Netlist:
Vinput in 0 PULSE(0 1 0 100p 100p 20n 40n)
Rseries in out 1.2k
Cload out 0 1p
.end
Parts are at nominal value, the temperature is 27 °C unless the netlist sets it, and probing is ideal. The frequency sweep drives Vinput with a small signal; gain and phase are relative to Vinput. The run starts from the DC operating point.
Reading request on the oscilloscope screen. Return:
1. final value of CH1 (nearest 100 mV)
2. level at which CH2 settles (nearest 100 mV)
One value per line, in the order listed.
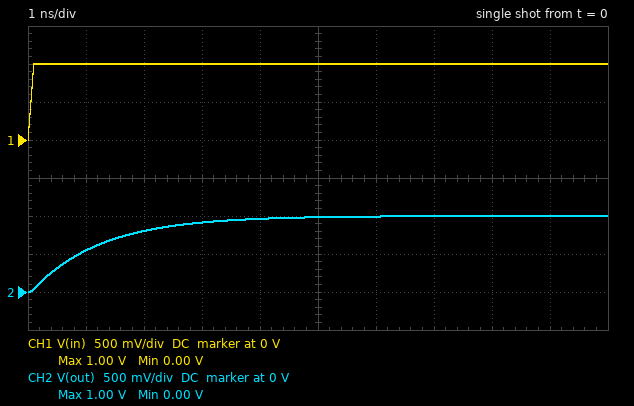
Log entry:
1.0 V
1.0 V
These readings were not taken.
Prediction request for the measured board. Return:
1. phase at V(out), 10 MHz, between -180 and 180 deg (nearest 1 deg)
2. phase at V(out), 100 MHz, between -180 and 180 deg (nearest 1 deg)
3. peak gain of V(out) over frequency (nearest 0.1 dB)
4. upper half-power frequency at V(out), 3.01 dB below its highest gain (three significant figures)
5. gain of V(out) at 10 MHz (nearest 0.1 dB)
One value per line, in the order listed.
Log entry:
-4 deg
-37 deg
0 dB
133 MHz
0 dB
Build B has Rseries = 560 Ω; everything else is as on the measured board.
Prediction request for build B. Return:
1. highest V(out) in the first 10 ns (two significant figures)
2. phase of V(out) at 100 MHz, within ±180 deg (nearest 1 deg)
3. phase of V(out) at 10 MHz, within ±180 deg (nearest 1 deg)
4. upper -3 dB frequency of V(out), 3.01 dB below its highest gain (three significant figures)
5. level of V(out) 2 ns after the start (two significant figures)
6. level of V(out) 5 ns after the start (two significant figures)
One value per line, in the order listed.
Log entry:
1.0 V
-19 deg
-2 deg
284 MHz
970 mV
1.0 V
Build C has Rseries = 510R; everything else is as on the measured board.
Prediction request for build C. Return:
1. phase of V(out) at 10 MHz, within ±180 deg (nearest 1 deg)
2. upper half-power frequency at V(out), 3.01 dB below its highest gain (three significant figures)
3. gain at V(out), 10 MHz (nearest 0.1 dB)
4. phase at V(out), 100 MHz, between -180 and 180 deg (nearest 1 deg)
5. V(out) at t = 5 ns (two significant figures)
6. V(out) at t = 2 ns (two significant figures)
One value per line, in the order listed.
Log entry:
-2 deg
312 MHz
0 dB
-18 deg
1.0 V
980 mV
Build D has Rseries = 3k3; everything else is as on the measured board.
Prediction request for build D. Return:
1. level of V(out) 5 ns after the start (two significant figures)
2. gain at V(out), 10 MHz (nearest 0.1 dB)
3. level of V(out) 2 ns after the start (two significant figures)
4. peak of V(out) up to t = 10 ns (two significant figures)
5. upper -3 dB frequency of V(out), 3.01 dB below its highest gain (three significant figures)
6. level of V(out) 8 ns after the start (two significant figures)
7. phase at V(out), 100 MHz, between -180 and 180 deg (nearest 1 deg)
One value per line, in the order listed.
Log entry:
780 mV
-0.2 dB
450 mV
950 mV
48.2 MHz
910 mV
-64 deg
